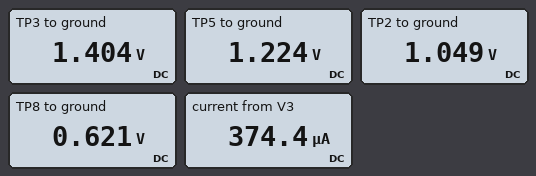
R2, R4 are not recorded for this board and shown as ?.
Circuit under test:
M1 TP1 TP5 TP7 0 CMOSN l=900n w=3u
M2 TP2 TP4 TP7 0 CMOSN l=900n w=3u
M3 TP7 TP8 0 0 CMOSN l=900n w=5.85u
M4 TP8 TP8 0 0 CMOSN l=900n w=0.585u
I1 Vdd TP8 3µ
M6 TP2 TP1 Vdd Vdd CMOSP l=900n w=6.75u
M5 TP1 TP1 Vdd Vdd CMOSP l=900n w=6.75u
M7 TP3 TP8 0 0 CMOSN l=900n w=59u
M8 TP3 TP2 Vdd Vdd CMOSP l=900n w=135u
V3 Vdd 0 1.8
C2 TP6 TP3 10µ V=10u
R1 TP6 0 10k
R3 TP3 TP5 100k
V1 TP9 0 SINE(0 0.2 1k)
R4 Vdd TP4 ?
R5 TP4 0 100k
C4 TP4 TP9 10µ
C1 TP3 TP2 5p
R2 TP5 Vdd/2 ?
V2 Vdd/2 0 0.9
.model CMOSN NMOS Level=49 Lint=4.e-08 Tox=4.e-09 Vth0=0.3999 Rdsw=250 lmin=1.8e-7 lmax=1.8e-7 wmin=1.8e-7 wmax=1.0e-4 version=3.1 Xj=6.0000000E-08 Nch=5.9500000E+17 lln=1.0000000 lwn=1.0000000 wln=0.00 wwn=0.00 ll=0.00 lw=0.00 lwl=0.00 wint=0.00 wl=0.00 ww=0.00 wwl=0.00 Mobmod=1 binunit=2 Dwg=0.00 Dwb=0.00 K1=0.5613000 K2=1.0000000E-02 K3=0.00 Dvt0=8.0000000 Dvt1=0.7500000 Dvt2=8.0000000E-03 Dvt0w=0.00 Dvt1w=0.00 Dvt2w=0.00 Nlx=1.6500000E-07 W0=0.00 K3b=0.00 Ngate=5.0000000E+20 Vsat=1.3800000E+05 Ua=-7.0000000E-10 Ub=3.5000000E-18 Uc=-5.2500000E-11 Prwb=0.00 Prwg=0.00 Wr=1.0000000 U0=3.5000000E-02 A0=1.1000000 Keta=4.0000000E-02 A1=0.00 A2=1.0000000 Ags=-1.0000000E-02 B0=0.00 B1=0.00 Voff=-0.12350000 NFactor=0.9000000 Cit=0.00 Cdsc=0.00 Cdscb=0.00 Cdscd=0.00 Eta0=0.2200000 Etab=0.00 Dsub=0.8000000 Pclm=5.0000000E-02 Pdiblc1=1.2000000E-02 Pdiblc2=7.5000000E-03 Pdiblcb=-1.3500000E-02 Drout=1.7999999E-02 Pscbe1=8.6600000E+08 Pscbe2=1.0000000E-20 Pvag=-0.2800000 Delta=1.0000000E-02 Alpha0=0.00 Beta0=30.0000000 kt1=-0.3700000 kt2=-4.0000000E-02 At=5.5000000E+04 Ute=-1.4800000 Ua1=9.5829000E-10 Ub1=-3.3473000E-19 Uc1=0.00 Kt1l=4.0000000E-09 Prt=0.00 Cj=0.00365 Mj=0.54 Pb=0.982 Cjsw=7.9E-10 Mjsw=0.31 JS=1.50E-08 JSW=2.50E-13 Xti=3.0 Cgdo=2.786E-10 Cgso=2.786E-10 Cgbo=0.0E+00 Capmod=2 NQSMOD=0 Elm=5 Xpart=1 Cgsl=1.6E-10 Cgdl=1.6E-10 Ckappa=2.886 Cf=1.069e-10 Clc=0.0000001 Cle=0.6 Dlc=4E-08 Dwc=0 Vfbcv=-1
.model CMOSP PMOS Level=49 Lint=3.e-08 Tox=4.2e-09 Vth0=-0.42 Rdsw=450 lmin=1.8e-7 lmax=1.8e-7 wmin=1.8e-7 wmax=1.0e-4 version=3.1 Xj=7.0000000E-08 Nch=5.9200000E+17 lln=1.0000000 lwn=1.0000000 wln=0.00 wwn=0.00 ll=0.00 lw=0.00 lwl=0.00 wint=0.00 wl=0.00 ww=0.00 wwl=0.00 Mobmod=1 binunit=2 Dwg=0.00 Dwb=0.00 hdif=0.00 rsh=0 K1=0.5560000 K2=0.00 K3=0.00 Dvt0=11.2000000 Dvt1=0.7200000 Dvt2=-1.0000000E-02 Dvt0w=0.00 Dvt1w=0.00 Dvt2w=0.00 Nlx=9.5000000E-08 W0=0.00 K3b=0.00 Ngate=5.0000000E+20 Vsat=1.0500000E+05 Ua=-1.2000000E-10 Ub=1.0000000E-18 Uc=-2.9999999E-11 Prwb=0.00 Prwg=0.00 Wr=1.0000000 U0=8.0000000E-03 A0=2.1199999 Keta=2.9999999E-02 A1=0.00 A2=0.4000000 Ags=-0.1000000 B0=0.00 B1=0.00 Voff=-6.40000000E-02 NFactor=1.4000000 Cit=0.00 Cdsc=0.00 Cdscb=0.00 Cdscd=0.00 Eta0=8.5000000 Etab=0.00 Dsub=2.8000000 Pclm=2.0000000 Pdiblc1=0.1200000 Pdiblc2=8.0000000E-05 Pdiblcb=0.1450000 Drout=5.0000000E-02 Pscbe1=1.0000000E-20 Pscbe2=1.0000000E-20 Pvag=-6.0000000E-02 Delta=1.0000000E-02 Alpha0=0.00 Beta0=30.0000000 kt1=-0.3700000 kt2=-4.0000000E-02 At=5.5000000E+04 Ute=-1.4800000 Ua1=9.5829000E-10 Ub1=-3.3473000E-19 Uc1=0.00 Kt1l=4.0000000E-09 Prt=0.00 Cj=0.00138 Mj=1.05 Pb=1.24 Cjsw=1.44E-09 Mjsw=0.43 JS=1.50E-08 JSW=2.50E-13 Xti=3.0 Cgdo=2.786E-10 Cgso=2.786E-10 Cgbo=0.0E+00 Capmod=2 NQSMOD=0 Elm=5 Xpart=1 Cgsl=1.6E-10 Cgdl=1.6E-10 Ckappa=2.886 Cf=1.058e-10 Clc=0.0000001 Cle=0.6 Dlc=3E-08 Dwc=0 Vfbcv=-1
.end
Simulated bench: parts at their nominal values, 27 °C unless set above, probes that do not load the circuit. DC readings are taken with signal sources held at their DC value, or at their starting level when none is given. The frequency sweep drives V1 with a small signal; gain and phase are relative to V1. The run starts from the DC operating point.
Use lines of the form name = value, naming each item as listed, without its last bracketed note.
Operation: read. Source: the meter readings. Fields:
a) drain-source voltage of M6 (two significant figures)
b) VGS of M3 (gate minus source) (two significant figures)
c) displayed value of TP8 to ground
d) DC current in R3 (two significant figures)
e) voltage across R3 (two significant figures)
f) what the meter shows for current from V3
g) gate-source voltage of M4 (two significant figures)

drain-source voltage of M6 = -750 mV
VGS of M3 (gate minus source) = 620 mV
displayed value of TP8 to ground = 0.621 V
DC current in R3 = 1.8 µA
voltage across R3 = 180 mV
what the meter shows for current from V3 = 374.4 µA
gate-source voltage of M4 = 620 mV
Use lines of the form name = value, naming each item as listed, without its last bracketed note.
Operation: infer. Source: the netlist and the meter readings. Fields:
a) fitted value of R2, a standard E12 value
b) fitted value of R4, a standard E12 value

fitted value of R2, a standard E12 value = 180 kΩ
fitted value of R4, a standard E12 value = 47 kΩ
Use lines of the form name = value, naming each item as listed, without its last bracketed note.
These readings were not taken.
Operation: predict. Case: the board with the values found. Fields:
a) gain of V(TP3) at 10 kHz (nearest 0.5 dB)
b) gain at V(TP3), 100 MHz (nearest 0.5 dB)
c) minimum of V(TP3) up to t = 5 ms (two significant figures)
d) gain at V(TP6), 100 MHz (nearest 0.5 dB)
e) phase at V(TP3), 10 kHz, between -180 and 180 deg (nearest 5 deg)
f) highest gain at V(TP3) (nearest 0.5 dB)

gain of V(TP3) at 10 kHz = 4.0 dB
gain at V(TP3), 100 MHz = -26.0 dB
minimum of V(TP3) up to t = 5 ms = 1.1 V
gain at V(TP6), 100 MHz = -26.0 dB
phase at V(TP3), 10 kHz, between -180 and 180 deg = 0 deg
highest gain at V(TP3) = 4.0 dB
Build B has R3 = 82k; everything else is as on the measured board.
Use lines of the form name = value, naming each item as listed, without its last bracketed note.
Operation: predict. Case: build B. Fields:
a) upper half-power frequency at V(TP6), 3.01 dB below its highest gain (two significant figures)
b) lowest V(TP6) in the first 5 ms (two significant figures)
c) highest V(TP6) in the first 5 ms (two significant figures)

upper half-power frequency at V(TP6), 3.01 dB below its highest gain = 2.9 MHz
lowest V(TP6) in the first 5 ms = -290 mV
highest V(TP6) in the first 5 ms = 290 mV
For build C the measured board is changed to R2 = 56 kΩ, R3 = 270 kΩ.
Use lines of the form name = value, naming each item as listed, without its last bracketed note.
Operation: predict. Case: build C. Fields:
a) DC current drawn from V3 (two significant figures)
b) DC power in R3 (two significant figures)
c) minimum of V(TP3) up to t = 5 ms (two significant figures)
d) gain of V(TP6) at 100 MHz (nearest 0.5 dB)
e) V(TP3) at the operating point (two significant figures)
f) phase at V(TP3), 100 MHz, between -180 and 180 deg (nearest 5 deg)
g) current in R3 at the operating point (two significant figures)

DC current drawn from V3 = 390 µA
DC power in R3 = 1.9 µW
minimum of V(TP3) up to t = 5 ms = 1.6 V
gain of V(TP6) at 100 MHz = -48.5 dB
V(TP3) at the operating point = 1.8 V
phase at V(TP3), 100 MHz, between -180 and 180 deg = 140 deg
current in R3 at the operating point = 2.6 µA
